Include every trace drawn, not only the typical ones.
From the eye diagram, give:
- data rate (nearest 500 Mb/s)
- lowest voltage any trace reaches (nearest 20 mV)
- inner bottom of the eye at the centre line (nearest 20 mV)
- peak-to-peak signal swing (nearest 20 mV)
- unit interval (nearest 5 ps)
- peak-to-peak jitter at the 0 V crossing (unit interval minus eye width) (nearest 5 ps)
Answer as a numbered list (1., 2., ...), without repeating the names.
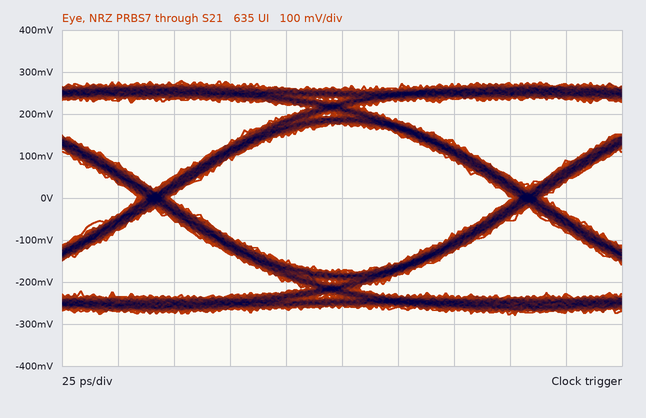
1. 6.0 Gb/s
2. -280 mV
3. -180 mV
4. 560 mV
5. 165 ps
6. 15 ps
